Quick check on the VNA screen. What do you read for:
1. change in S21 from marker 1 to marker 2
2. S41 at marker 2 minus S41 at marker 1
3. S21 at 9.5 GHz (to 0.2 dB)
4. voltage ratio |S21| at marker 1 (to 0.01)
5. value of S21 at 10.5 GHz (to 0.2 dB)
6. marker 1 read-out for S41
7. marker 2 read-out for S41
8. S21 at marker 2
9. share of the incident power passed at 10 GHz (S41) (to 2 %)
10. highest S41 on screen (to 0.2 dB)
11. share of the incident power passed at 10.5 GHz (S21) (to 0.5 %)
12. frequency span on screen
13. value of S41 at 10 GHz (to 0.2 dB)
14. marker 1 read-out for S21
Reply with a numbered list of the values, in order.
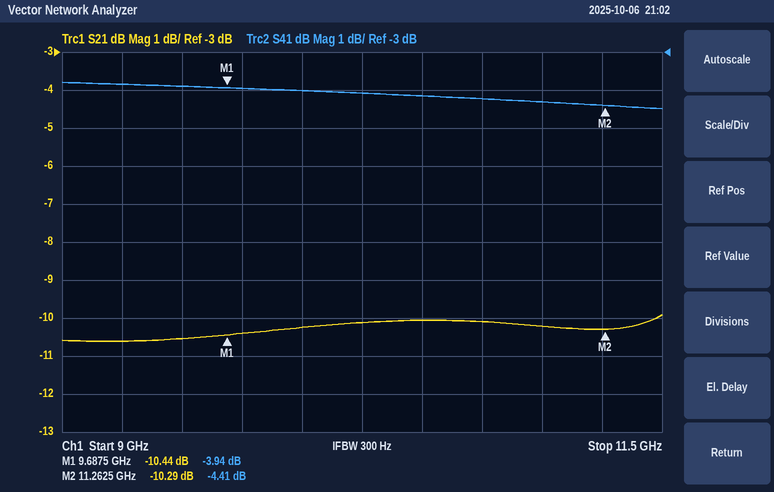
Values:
1. 0.15 dB
2. -0.47 dB
3. -10.6 dB
4. 0.30
5. -10.0 dB
6. -3.94 dB
7. -4.41 dB
8. -10.29 dB
9. 40 %
10. -3.8 dB
11. 10.0 %
12. 2.5 GHz
13. -4.0 dB
14. -10.44 dB
